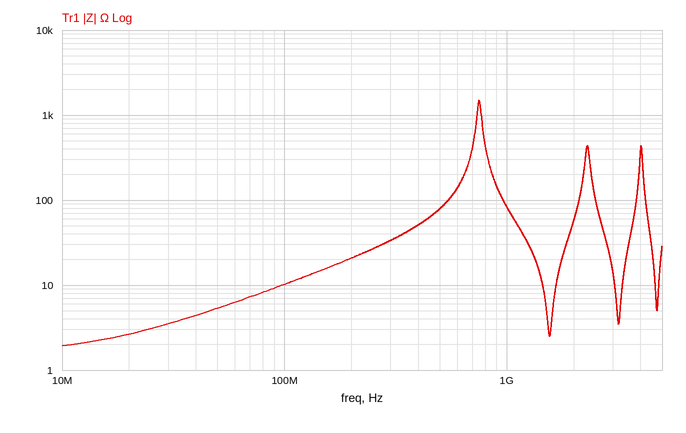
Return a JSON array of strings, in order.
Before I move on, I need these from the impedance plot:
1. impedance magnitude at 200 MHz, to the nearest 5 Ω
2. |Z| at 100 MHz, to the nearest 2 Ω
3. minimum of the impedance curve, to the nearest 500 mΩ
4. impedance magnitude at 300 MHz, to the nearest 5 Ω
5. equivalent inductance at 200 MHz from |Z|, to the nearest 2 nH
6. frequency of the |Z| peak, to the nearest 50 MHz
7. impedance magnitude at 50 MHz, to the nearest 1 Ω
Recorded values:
["20 Ω", "10 Ω", "2.0 Ω", "35 Ω", "16 nH", "750 MHz", "5 Ω"]
